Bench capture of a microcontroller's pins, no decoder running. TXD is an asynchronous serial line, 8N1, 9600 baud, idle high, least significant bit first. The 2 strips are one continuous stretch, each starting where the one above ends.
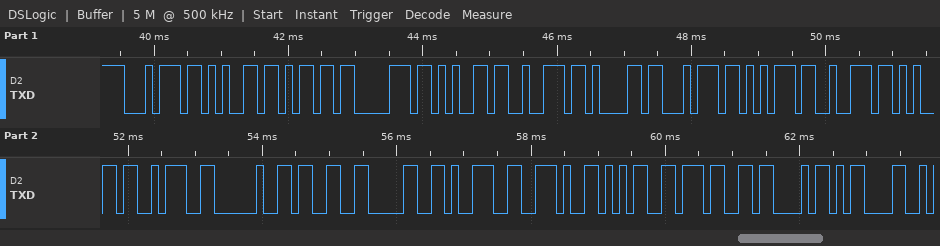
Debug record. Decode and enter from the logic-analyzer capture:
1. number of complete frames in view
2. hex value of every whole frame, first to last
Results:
21
0x74 0x65 0x6D 0x70 0x65 0x72 0x61 0x74 0x75 0x72 0x65 0x3A 0x20 0x33 0x30 0x39 0x2E 0x35 0x37 0x43 0x0D
